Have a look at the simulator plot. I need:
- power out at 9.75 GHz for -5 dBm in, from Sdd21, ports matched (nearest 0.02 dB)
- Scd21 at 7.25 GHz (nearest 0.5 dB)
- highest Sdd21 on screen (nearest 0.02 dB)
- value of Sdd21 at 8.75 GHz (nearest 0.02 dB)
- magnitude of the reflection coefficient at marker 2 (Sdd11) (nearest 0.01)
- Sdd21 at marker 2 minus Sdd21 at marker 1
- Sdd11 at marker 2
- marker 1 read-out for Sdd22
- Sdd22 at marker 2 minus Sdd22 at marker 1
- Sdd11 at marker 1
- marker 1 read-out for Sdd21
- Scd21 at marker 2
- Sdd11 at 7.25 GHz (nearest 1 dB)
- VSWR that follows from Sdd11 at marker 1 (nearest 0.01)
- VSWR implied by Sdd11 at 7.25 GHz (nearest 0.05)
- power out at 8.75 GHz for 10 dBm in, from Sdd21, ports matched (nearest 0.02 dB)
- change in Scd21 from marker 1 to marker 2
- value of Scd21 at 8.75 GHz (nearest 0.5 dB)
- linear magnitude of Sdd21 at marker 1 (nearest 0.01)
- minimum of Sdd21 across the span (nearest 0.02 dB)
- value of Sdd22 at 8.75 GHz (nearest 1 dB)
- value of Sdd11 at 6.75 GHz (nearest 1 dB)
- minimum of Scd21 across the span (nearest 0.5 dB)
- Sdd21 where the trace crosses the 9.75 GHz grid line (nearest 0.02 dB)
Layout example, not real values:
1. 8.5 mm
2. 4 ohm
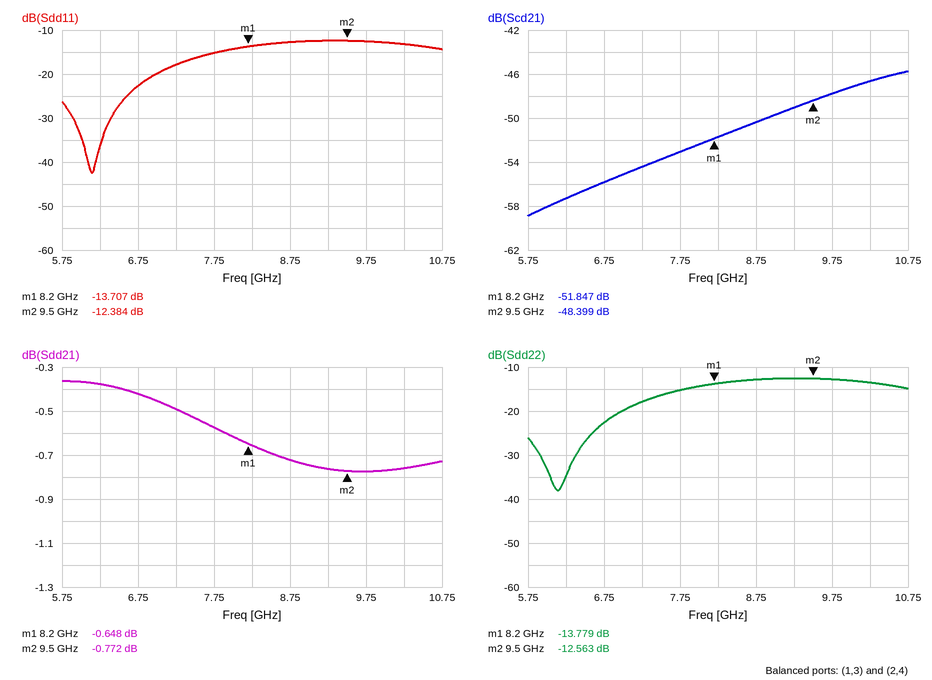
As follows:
1. -5.78 dBm
2. -54.5 dB
3. -0.36 dB
4. -0.72 dB
5. 0.24
6. -0.124 dB
7. -12.384 dB
8. -13.779 dB
9. 1.216 dB
10. -13.707 dB
11. -0.648 dB
12. -48.399 dB
13. -18 dB
14. 1.52
15. 1.30
16. 9.28 dBm
17. 3.448 dB
18. -50.5 dB
19. 0.93
20. -0.78 dB
21. -13 dB
22. -23 dB
23. -59.0 dB
24. -0.78 dB
